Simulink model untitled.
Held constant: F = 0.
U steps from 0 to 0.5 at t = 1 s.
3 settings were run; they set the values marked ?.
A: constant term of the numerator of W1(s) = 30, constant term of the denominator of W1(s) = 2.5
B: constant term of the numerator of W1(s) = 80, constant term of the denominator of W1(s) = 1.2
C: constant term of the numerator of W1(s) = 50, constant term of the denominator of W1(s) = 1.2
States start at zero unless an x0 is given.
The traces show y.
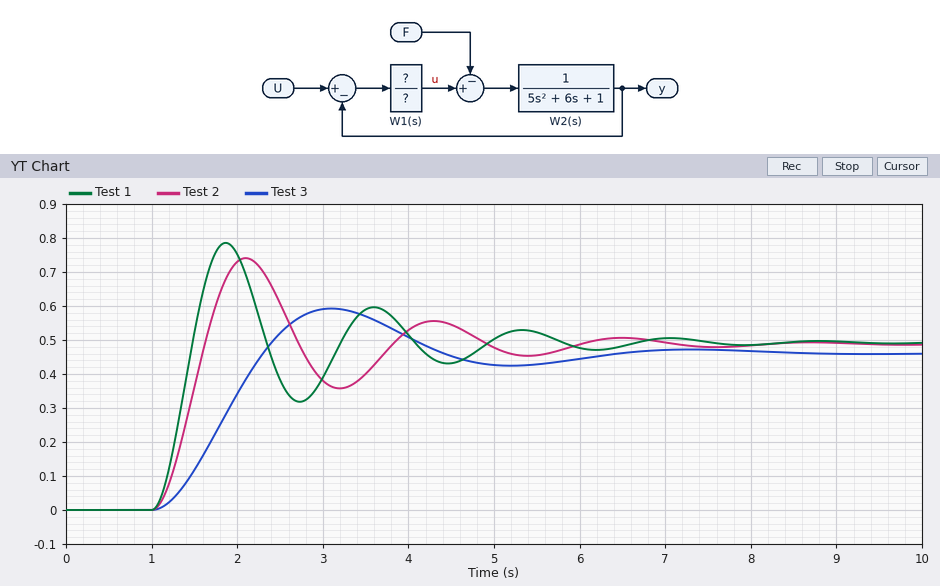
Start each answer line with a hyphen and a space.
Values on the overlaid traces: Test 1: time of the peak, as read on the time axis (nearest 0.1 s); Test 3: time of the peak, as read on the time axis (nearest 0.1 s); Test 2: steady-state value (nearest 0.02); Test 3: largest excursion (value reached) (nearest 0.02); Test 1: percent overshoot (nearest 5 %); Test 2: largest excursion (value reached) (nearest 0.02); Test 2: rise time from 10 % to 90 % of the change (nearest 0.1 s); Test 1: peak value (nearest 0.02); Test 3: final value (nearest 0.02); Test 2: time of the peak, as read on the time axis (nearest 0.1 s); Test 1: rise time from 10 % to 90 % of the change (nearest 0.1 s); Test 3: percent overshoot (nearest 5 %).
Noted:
- 1.9 s
- 3.1 s
- 0.48
- 0.60
- 60 %
- 0.74
- 0.4 s
- 0.78
- 0.46
- 2.1 s
- 0.3 s
- 30 %
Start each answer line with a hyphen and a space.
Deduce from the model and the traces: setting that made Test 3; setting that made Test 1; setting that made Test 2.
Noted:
- A
- B
- C
